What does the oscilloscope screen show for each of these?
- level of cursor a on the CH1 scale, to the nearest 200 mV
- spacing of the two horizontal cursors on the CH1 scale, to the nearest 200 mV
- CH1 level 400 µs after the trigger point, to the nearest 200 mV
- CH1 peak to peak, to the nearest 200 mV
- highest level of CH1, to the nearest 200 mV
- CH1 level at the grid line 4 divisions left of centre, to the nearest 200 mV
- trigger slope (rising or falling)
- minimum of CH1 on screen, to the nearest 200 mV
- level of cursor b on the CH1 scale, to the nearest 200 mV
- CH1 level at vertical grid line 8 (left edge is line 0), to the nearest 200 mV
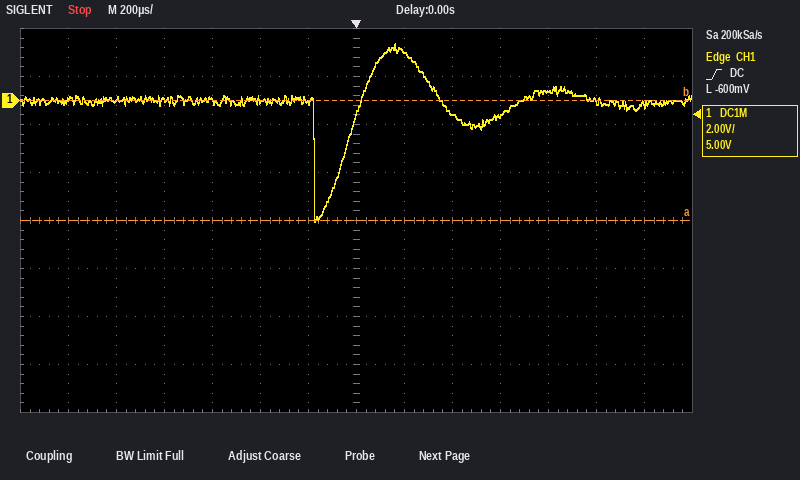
-5.0 V
5.0 V
-600 mV
7.4 V
2.4 V
0.0 V
rising
-5.0 V
0.0 V
2.0 V
